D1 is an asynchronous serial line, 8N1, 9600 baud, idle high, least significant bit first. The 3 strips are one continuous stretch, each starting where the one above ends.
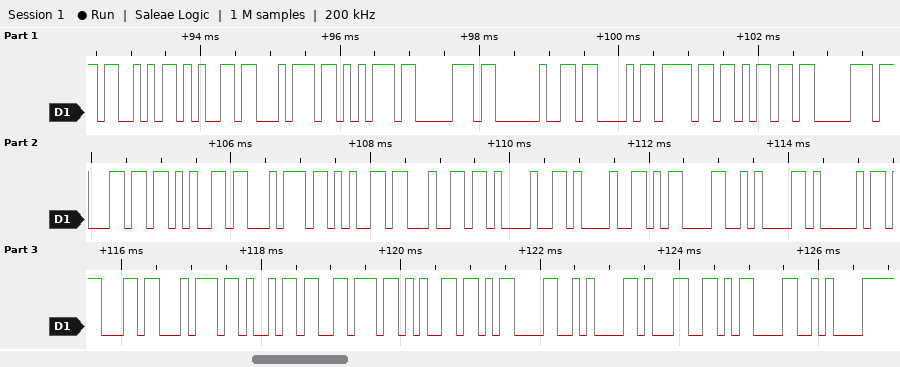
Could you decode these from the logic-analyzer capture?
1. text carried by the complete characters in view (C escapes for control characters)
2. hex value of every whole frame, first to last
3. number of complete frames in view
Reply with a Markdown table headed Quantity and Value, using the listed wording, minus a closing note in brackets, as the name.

| Quantity | Value |
|---|---|
| text carried by the complete characters in view | "Setup Completed!!\r\nActive\r\n1\r\n" |
| hex value of every whole frame, first to last | 0x53 0x65 0x74 0x75 0x70 0x20 0x43 0x6F 0x6D 0x70 0x6C 0x65 0x74 0x65 0x64 0x21 0x21 0x0D 0x0A 0x41 0x63 0x74 0x69 0x76 0x65 0x0D 0x0A 0x31 0x0D 0x0A |
| number of complete frames in view | 30 |
